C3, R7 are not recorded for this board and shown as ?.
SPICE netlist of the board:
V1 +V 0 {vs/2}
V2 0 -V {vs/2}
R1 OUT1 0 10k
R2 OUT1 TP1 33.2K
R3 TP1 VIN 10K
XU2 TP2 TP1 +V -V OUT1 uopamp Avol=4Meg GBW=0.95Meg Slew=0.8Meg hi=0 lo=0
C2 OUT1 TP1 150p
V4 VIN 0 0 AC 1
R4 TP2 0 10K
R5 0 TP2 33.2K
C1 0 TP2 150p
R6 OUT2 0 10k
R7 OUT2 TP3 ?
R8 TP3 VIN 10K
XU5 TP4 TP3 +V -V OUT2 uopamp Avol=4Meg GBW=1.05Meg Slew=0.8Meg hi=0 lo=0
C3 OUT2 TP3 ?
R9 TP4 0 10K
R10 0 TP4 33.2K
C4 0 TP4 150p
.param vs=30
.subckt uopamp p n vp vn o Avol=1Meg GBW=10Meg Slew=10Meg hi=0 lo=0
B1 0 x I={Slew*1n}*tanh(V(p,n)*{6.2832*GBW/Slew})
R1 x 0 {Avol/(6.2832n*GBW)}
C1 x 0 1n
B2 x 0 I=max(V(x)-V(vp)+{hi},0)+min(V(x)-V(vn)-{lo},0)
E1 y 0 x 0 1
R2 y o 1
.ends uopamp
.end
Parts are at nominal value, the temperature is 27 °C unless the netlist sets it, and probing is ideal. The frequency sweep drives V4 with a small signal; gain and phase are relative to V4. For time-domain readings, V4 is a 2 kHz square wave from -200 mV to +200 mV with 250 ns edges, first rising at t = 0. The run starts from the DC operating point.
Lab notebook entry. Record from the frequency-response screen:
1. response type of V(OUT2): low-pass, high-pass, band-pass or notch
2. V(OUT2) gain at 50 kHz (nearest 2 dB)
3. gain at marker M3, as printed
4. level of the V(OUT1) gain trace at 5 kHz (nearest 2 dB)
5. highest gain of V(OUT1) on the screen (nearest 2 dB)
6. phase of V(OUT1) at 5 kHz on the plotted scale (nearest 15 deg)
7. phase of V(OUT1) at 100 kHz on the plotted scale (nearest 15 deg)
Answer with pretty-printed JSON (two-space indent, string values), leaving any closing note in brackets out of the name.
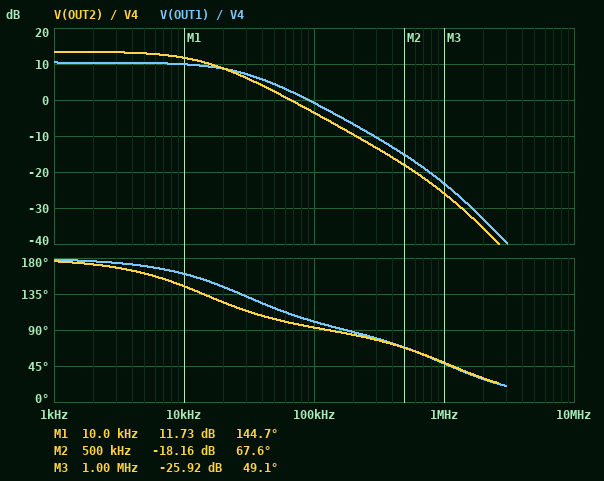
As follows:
{
  "response type of V(OUT2): low-pass, high-pass, band-pass or notch": "low-pass",
  "V(OUT2) gain at 50 kHz": "2 dB",
  "gain at marker M3, as printed": "-25.92 dB",
  "level of the V(OUT1) gain trace at 5 kHz": "10 dB",
  "highest gain of V(OUT1) on the screen": "10 dB",
  "phase of V(OUT1) at 5 kHz on the plotted scale": "165 deg",
  "phase of V(OUT1) at 100 kHz on the plotted scale": "105 deg"
}
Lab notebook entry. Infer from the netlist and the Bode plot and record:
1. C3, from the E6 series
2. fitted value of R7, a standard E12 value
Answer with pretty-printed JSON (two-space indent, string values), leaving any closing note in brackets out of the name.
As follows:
{
  "C3, from the E6 series": "220 pF",
  "fitted value of R7, a standard E12 value": "47 kΩ"
}
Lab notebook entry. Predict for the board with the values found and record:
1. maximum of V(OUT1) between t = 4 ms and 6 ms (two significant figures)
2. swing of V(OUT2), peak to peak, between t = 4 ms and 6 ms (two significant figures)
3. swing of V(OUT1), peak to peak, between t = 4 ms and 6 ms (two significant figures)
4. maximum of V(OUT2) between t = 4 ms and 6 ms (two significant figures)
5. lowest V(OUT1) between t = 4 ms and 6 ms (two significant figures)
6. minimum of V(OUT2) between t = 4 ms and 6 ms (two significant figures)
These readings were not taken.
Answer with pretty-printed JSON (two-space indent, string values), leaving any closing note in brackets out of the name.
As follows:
{
  "maximum of V(OUT1) between t = 4 ms and 6 ms": "660 mV",
  "swing of V(OUT2), peak to peak, between t = 4 ms and 6 ms": "1.9 V",
  "swing of V(OUT1), peak to peak, between t = 4 ms and 6 ms": "1.3 V",
  "maximum of V(OUT2) between t = 4 ms and 6 ms": "940 mV",
  "lowest V(OUT1) between t = 4 ms and 6 ms": "-660 mV",
  "minimum of V(OUT2) between t = 4 ms and 6 ms": "-940 mV"
}
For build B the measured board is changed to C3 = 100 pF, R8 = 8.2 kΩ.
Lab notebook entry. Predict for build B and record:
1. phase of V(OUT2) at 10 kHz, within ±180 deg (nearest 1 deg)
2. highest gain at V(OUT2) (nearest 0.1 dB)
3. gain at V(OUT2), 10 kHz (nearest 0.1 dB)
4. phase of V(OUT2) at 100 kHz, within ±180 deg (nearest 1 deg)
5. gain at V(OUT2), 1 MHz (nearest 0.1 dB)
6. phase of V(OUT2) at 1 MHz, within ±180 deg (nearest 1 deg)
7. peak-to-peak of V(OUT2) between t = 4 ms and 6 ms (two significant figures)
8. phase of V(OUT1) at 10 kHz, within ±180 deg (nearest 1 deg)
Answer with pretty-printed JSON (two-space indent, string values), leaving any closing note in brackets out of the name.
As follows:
{
  "phase of V(OUT2) at 10 kHz, within ±180 deg": "160 deg",
  "highest gain at V(OUT2)": "15.2 dB",
  "gain at V(OUT2), 10 kHz": "14.7 dB",
  "phase of V(OUT2) at 100 kHz, within ±180 deg": "101 deg",
  "gain at V(OUT2), 1 MHz": "-17.9 dB",
  "phase of V(OUT2) at 1 MHz, within ±180 deg": "53 deg",
  "peak-to-peak of V(OUT2) between t = 4 ms and 6 ms": "2.3 V",
  "phase of V(OUT1) at 10 kHz, within ±180 deg": "160 deg"
}
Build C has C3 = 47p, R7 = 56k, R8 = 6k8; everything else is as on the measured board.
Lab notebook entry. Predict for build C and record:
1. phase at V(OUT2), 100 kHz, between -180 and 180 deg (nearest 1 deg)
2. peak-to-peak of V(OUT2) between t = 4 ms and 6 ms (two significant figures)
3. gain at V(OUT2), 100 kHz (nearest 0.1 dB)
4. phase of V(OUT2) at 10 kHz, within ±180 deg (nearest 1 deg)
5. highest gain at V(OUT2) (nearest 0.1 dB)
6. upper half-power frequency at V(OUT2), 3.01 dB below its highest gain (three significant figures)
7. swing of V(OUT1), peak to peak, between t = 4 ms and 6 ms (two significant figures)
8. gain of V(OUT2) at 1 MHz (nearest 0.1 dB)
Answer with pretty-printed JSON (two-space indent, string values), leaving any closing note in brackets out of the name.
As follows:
{
  "phase at V(OUT2), 100 kHz, between -180 and 180 deg": "108 deg",
  "peak-to-peak of V(OUT2) between t = 4 ms and 6 ms": "3.3 V",
  "gain at V(OUT2), 100 kHz": "9.8 dB",
  "phase of V(OUT2) at 10 kHz, within ±180 deg": "166 deg",
  "highest gain at V(OUT2)": "18.3 dB",
  "upper half-power frequency at V(OUT2), 3.01 dB below its highest gain": "40.5 kHz",
  "swing of V(OUT1), peak to peak, between t = 4 ms and 6 ms": "1.3 V",
  "gain of V(OUT2) at 1 MHz": "-11.0 dB"
}
